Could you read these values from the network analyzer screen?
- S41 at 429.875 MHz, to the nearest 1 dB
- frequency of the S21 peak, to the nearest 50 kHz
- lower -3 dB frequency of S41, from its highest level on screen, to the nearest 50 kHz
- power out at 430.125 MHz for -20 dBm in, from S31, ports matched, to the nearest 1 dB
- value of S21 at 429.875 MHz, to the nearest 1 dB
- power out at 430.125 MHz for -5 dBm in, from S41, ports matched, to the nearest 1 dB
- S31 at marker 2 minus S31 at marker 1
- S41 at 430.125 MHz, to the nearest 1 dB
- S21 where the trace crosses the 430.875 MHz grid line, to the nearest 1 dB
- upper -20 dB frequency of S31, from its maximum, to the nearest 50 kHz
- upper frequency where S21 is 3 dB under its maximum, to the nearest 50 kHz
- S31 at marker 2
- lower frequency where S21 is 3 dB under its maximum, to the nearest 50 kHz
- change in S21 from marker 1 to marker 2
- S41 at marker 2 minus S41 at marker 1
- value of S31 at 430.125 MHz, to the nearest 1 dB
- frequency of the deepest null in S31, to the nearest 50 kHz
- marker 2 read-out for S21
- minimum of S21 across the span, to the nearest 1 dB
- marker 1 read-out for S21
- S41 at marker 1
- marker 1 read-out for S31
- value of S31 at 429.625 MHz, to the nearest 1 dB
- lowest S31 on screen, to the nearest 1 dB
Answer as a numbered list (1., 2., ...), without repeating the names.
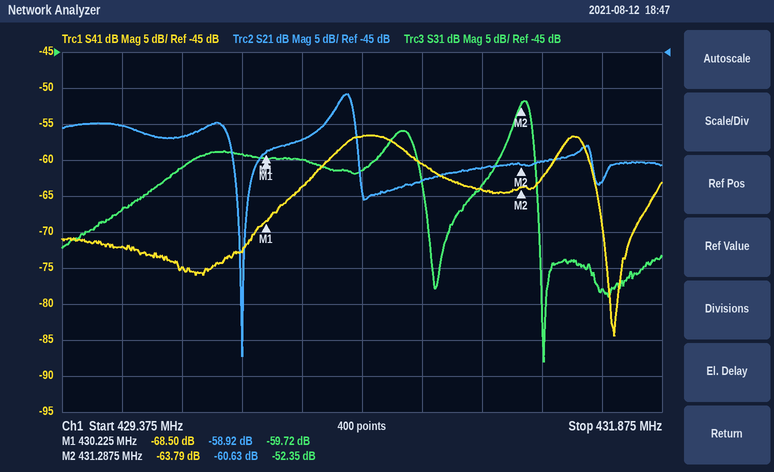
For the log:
1. -75 dB
2. 430.55 MHz
3. 430.50 MHz
4. -79 dBm
5. -57 dB
6. -78 dBm
7. 7.37 dB
8. -73 dB
9. -63 dB
10. 431.35 MHz
11. 430.60 MHz
12. -52.35 dB
13. 430.50 MHz
14. -1.71 dB
15. 4.71 dB
16. -59 dB
17. 431.40 MHz
18. -60.63 dB
19. -87 dB
20. -58.92 dB
21. -68.50 dB
22. -59.72 dB
23. -67 dB
24. -88 dB
